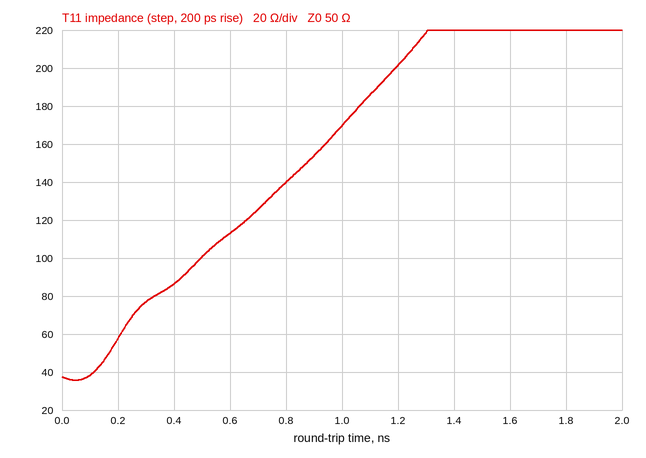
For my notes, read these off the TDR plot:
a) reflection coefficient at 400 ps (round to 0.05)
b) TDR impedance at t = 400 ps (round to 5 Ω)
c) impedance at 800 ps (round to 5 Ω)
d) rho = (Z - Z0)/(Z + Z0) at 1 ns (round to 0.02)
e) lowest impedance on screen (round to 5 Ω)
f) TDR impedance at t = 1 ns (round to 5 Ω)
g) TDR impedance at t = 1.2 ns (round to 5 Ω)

+0.25
85 Ω
140 Ω
+0.54
35 Ω
170 Ω
200 Ω
